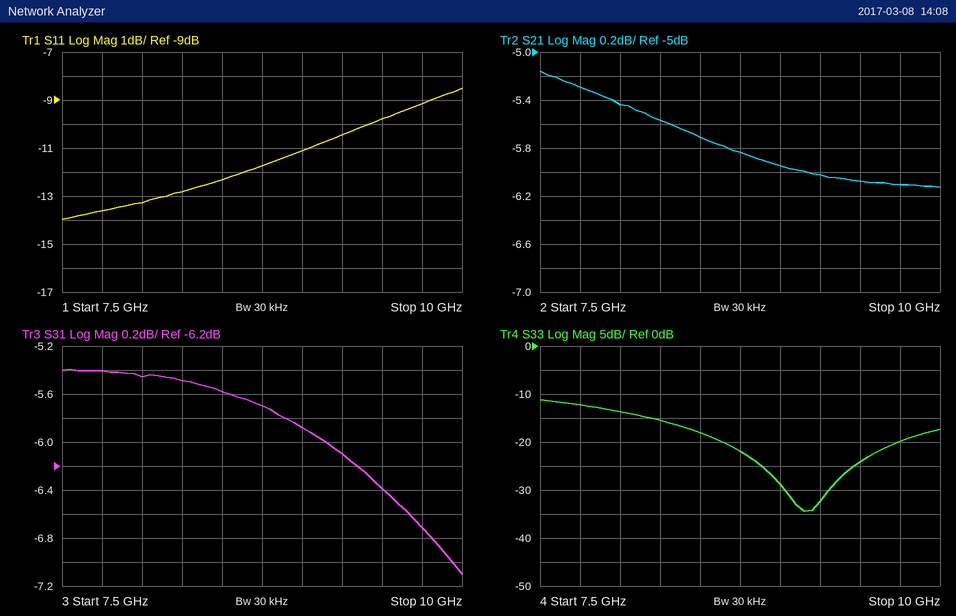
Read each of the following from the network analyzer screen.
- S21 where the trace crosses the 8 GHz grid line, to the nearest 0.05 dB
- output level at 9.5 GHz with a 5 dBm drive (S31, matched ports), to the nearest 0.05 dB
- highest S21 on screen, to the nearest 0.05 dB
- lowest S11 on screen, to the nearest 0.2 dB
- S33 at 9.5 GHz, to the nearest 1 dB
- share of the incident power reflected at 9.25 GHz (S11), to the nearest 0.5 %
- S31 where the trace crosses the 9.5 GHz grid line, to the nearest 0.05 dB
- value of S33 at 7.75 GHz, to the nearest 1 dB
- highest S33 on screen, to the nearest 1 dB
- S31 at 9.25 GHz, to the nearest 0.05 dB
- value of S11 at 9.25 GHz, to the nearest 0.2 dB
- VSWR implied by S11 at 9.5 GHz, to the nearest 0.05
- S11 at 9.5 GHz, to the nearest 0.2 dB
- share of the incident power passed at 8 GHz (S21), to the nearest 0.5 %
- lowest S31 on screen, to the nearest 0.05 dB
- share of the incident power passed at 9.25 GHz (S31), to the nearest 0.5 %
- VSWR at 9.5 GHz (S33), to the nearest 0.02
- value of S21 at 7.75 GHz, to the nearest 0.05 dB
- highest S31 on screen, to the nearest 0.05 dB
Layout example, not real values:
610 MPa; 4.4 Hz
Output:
-5.45 dB; -1.40 dBm; -5.15 dB; -14.0 dB; -24 dB; 9.0 %; -6.40 dB; -12 dB; -11 dB; -6.10 dB; -10.4 dB; 1.95; -9.8 dB; 28.5 %; -7.10 dB; 24.5 %; 1.14; -5.30 dB; -5.40 dB
